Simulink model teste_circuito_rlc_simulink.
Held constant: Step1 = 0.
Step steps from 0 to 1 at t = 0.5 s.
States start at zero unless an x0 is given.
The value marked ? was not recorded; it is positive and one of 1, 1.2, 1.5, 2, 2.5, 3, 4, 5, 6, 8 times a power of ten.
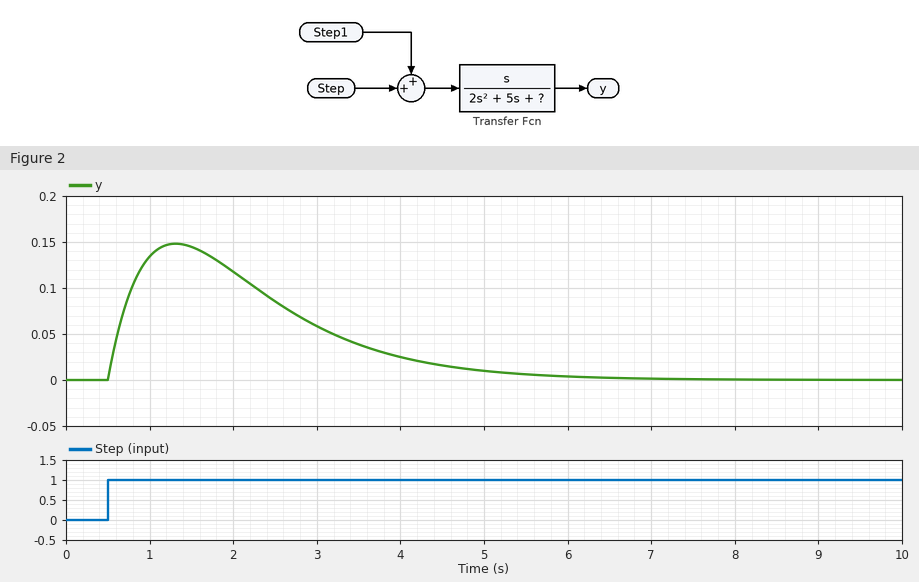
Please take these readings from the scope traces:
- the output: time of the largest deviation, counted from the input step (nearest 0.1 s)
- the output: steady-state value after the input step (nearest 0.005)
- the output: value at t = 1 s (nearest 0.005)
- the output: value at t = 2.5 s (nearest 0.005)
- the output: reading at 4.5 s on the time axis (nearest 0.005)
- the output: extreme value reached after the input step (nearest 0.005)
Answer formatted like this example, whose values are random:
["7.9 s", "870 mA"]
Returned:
["0.8 s", "0.000", "0.135", "0.085", "0.015", "0.150"]
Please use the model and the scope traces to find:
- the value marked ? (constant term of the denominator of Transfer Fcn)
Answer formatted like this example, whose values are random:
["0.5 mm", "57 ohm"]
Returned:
["3"]
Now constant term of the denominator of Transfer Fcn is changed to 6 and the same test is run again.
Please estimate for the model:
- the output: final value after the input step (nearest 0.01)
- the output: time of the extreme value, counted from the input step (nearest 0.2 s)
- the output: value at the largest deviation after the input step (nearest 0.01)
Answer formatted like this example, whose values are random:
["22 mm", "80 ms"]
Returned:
["0.00", "0.6 s", "0.13"]
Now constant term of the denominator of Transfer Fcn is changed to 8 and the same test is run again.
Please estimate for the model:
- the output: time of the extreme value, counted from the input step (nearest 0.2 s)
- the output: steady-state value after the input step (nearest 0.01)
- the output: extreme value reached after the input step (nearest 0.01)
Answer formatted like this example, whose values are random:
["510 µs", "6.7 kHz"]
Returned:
["0.6 s", "0.00", "0.12"]
